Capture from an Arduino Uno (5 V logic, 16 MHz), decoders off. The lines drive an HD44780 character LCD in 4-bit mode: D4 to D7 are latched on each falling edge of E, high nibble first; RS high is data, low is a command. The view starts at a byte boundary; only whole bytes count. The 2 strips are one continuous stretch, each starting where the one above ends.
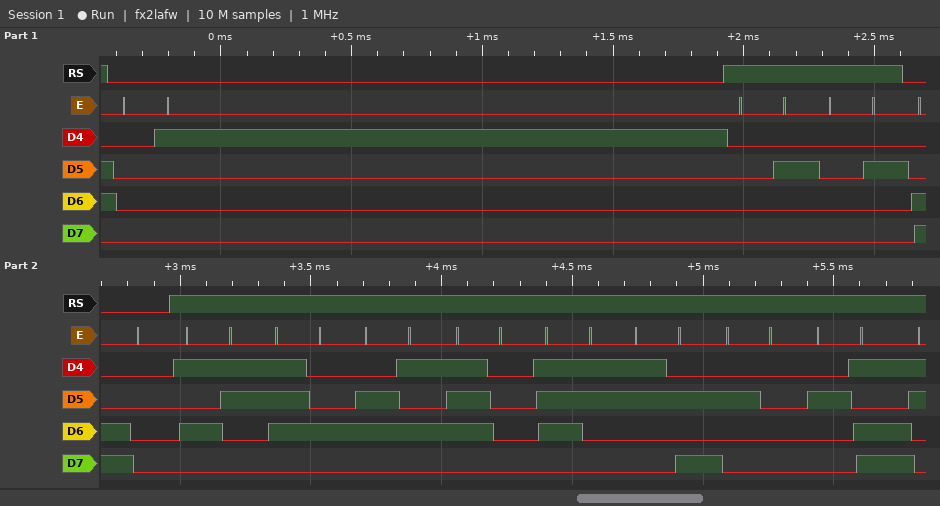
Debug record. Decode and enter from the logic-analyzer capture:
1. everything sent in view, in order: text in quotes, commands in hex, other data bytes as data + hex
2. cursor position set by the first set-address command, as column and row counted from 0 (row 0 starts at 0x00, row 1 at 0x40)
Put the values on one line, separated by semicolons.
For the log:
0x01 data 02 02 0xC0 "Steps: -"; column 0, row 1
